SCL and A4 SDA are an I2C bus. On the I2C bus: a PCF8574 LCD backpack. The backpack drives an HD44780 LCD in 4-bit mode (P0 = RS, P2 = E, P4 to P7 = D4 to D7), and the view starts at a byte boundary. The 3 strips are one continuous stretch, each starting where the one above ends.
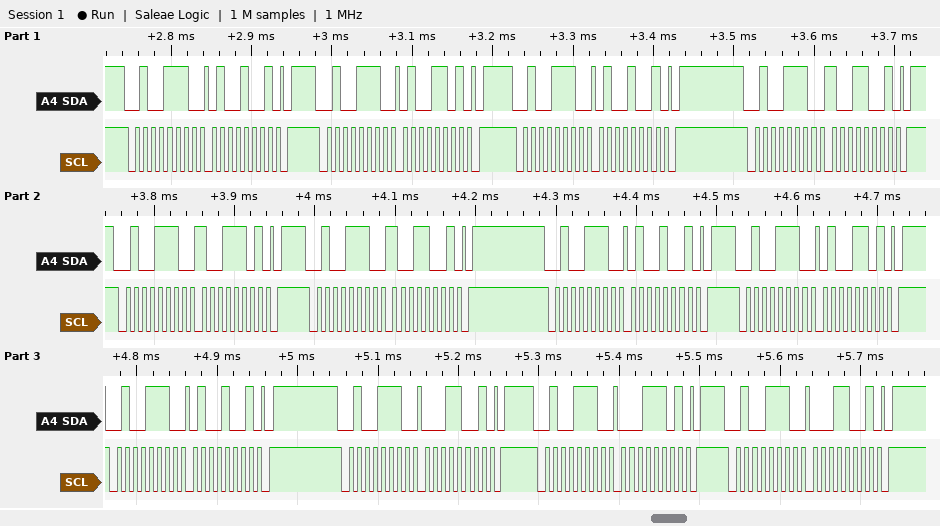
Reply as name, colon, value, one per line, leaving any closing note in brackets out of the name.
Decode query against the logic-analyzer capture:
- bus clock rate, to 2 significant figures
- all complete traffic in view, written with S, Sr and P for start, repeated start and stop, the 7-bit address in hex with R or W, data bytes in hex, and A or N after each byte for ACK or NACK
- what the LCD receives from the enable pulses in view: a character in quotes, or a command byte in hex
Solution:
bus clock rate, to 2 significant figures: 100 kHz
all complete traffic in view, written with S, Sr and P for start, repeated start and stop, the 7-bit address in hex with R or W, data bytes in hex, and A or N after each byte for ACK or NACK: S 27W A 49 A P S 27W A 4D A P S 27W A 49 A P S 27W A 99 A P S 27W A 9D A P S 27W A 99 A P S 27W A 49 A P S 27W A 4D A P S 27W A 49 A P S 27W A 19 A P S 27W A 1D A P S 27W A 19 A P
what the LCD receives from the enable pulses in view: a character in quotes, or a command byte in hex: 'I' 'A'
